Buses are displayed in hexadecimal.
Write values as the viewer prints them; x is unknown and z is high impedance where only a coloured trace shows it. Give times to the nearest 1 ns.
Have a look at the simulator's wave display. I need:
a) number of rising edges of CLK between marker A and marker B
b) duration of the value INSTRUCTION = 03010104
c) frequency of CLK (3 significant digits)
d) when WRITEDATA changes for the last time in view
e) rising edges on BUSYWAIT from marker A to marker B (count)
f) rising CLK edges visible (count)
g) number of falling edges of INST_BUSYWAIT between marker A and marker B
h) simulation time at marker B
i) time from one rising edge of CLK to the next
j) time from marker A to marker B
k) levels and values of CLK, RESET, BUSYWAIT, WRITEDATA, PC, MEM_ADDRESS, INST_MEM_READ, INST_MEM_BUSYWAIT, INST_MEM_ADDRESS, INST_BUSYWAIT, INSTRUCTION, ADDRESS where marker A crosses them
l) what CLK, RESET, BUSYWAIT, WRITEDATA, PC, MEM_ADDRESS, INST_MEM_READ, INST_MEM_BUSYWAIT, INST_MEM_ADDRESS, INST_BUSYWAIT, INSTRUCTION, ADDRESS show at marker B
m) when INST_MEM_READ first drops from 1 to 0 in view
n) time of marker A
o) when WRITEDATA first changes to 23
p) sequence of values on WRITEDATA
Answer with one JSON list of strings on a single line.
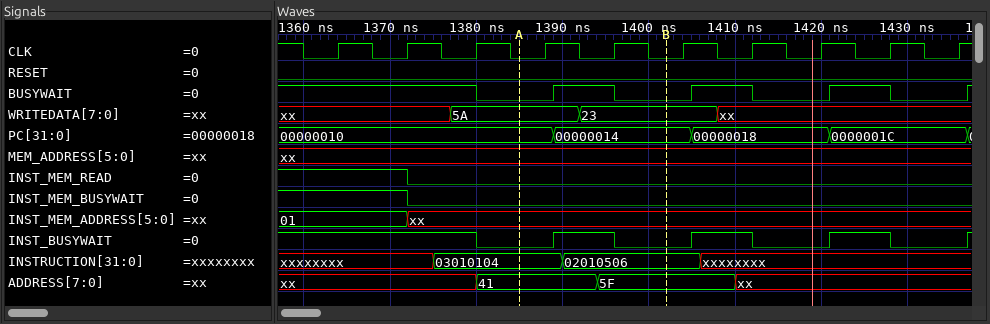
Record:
["2", "15 ns", "125 MHz", "1408 ns", "1", "10", "1", "1402 ns", "8 ns", "17 ns", "CLK=0, RESET=0, BUSYWAIT=0, WRITEDATA=5A, PC=00000010, MEM_ADDRESS=xx, INST_MEM_READ=0, INST_MEM_BUSYWAIT=0, INST_MEM_ADDRESS=xx, INST_BUSYWAIT=0, INSTRUCTION=03010104, ADDRESS=41", "CLK=0, RESET=0, BUSYWAIT=0, WRITEDATA=23, PC=00000014, MEM_ADDRESS=xx, INST_MEM_READ=0, INST_MEM_BUSYWAIT=0, INST_MEM_ADDRESS=xx, INST_BUSYWAIT=0, INSTRUCTION=02010506, ADDRESS=5F", "1372 ns", "1385 ns", "1392 ns", "xx, 5A, 23, xx"]
